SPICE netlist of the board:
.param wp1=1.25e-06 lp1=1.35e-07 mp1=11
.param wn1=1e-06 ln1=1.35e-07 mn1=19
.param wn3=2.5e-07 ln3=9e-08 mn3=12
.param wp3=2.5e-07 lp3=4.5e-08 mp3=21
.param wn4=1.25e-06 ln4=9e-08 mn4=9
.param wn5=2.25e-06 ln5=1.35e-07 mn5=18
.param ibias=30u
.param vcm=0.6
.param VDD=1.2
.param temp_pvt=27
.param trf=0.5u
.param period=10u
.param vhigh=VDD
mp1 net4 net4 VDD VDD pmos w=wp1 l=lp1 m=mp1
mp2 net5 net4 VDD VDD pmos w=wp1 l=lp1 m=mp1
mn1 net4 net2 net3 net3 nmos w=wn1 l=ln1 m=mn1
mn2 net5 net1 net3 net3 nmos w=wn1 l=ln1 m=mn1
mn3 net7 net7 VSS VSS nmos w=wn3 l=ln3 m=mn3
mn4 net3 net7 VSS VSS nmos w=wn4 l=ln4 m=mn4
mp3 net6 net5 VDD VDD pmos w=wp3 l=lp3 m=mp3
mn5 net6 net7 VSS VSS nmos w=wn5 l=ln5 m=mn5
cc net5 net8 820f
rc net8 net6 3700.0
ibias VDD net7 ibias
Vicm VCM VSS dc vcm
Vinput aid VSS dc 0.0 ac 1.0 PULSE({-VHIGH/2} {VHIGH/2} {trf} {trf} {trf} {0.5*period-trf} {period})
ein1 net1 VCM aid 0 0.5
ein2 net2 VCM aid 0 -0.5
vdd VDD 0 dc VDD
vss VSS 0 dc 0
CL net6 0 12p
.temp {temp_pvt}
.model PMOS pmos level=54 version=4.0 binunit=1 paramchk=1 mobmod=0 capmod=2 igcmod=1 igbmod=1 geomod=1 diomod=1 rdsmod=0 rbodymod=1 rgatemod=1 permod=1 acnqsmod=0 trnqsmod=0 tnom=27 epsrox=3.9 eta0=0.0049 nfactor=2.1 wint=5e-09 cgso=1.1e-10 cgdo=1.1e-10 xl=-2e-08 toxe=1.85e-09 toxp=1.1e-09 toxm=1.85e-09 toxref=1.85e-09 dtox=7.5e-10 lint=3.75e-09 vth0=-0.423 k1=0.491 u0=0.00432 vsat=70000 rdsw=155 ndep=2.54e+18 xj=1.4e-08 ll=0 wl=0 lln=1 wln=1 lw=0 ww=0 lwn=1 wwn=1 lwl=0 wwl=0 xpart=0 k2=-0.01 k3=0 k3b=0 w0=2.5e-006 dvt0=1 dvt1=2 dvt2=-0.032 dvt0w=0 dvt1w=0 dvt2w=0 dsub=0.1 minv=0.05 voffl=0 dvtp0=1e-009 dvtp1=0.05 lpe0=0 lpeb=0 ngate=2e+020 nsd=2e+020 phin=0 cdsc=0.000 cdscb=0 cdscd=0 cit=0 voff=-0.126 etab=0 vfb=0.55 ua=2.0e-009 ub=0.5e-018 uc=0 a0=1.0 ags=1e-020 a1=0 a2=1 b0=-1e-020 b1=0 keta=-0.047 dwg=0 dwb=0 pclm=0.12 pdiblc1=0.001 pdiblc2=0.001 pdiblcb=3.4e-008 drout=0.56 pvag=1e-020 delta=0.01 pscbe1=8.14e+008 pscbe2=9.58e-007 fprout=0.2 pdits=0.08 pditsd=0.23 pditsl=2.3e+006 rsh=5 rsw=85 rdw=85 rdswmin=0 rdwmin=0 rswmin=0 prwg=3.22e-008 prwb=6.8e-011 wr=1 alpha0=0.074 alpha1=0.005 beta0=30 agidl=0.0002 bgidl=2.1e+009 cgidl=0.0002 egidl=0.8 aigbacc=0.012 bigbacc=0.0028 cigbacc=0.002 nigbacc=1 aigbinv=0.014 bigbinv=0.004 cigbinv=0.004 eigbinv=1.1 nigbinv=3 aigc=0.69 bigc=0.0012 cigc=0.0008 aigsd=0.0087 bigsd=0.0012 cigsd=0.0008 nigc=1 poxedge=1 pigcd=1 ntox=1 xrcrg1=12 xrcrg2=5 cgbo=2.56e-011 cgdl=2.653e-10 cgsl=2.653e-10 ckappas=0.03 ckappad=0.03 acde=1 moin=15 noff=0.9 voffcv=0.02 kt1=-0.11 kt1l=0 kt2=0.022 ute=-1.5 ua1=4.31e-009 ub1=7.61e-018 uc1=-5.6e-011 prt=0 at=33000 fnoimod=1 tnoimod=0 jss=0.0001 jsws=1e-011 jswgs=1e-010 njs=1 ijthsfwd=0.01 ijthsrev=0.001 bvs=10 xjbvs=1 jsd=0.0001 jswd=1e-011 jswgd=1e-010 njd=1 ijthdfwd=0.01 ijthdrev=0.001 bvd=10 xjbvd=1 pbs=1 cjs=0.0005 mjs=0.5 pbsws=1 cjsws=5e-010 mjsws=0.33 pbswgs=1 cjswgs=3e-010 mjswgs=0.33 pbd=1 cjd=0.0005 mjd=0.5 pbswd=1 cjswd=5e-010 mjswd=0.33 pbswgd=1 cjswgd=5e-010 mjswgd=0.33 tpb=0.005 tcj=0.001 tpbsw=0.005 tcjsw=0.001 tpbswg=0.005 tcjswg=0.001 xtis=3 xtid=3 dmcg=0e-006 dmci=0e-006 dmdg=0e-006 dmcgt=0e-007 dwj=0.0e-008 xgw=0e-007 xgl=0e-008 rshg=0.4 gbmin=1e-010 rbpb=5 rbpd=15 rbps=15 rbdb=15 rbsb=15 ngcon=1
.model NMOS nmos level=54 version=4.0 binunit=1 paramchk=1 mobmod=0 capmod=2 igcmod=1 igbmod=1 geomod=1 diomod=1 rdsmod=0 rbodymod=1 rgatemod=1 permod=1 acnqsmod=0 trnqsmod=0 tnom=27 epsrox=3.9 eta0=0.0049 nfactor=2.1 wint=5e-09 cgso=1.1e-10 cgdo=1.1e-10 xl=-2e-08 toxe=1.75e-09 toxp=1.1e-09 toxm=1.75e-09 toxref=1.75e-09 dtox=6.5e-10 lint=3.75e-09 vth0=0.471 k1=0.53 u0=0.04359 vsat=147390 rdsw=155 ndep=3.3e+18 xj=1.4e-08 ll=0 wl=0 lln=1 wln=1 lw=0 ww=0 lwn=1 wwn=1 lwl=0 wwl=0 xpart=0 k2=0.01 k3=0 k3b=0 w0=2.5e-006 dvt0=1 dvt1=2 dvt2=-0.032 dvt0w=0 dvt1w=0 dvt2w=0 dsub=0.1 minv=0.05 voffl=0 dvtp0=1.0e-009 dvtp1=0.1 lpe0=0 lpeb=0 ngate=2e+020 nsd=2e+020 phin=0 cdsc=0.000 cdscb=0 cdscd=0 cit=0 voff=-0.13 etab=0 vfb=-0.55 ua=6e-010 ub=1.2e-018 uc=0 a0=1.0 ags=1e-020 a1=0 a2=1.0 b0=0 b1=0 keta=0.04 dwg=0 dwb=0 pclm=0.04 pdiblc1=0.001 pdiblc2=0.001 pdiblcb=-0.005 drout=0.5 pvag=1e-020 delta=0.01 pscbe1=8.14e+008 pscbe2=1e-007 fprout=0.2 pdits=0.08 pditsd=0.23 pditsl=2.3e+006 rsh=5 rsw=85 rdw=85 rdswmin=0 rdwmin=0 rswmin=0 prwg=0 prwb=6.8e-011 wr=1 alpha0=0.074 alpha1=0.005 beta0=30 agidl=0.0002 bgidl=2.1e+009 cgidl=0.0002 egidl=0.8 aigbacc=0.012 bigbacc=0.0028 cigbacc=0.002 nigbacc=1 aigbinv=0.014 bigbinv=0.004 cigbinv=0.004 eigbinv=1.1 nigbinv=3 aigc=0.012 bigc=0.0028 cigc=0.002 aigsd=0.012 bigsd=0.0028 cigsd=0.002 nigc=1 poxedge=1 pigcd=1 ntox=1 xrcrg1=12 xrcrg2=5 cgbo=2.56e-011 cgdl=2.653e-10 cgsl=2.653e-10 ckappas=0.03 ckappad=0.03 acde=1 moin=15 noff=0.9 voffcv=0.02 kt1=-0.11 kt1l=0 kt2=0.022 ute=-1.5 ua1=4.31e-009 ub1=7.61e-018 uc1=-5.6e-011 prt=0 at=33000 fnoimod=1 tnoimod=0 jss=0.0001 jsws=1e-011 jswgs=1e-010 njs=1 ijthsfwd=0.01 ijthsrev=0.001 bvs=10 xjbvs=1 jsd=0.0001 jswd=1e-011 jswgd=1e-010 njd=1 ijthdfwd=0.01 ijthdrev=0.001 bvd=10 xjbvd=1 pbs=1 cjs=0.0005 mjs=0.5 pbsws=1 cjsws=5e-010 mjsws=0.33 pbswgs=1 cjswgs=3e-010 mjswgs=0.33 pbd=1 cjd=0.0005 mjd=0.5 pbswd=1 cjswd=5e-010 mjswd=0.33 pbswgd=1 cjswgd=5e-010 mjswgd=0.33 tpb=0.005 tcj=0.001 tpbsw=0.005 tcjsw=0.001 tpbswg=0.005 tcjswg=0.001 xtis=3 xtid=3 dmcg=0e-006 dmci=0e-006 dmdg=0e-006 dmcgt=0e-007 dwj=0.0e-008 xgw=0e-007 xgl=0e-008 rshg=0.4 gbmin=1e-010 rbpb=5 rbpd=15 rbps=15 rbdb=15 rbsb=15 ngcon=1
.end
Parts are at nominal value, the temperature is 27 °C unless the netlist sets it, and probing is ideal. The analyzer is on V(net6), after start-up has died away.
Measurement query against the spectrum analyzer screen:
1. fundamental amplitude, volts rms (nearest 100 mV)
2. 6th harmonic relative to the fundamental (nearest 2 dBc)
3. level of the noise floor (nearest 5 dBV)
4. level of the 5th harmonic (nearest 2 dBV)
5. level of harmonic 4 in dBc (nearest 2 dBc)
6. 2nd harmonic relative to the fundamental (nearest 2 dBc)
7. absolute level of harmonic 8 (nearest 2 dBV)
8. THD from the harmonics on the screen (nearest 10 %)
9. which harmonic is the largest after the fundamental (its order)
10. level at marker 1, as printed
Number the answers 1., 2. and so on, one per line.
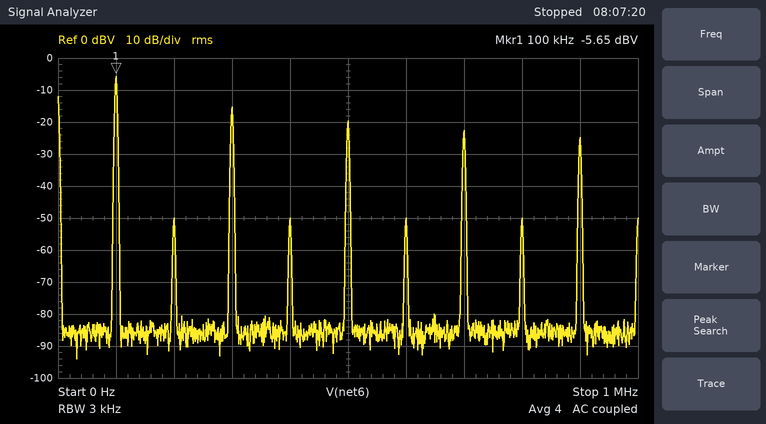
1. 500 mV
2. -44 dBc
3. -85 dBV
4. -20 dBV
5. -44 dBc
6. -44 dBc
7. -50 dBV
8. 40 %
9. 3
10. -5.65 dBV
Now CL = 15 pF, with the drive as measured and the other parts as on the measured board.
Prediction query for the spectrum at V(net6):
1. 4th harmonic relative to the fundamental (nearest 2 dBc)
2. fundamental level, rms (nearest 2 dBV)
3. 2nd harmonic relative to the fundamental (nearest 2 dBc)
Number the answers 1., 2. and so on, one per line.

1. -42 dBc
2. -6 dBV
3. -42 dBc
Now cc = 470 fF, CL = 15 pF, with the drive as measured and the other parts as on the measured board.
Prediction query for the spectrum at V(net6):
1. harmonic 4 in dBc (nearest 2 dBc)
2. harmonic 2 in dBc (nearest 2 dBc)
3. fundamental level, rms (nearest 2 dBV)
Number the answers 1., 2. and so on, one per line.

1. -42 dBc
2. -42 dBc
3. -6 dBV
